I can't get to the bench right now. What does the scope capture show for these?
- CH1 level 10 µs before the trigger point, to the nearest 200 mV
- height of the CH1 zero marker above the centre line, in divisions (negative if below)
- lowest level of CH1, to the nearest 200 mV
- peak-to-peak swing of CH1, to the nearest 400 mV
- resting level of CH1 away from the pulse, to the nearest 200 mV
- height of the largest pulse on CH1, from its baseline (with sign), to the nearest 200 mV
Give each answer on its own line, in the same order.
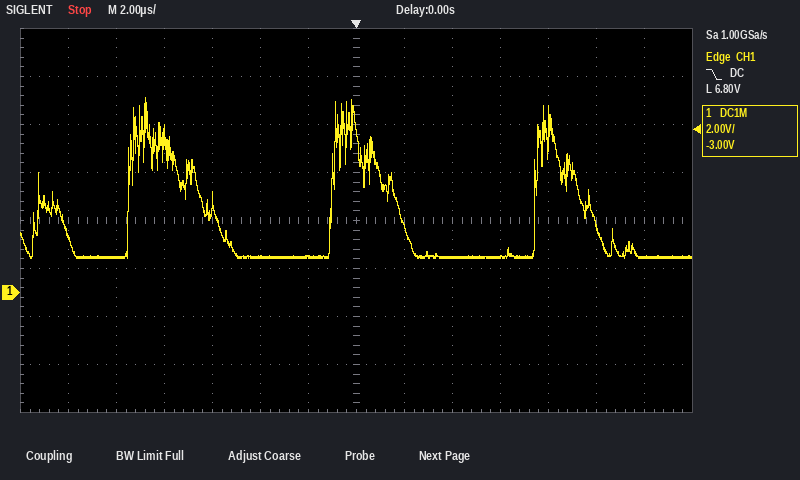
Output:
1.4 V
-1.5 div
1.4 V
6.8 V
1.4 V
+6.6 V
